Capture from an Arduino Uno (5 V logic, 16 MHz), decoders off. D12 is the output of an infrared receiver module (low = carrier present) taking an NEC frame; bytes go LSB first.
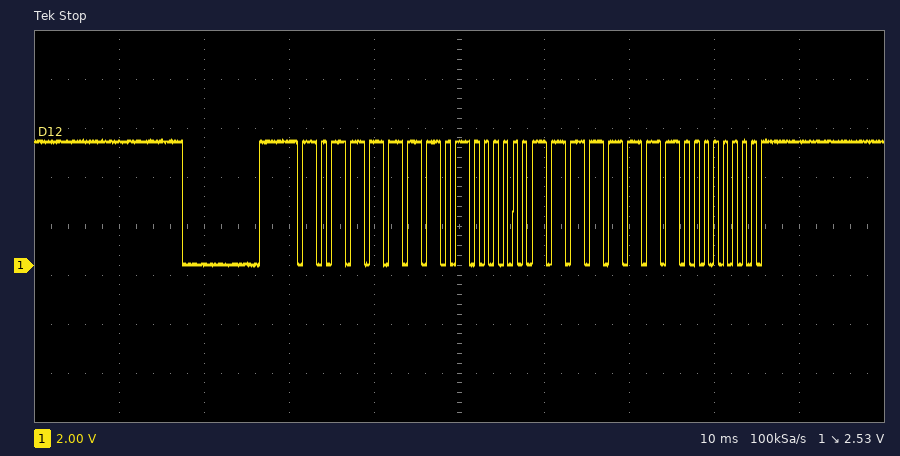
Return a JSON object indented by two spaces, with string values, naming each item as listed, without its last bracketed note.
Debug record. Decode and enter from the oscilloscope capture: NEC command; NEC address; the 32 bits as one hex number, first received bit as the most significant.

{
  "NEC command": "0xFF",
  "NEC address": "0xFD",
  "the 32 bits as one hex number, first received bit as the most significant": "0xBF40FF00"
}
